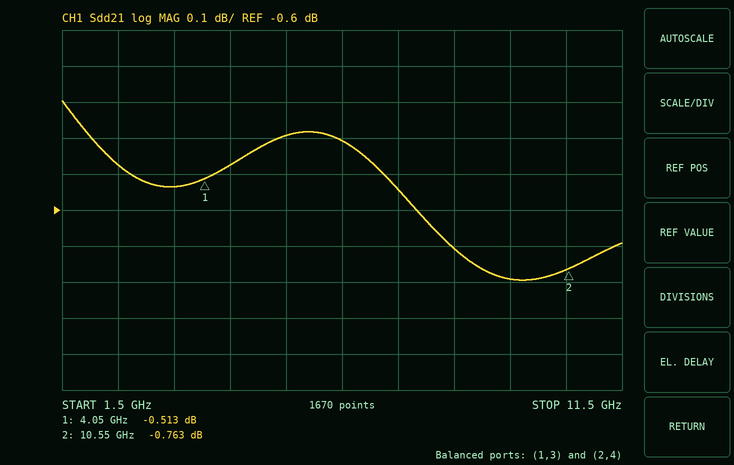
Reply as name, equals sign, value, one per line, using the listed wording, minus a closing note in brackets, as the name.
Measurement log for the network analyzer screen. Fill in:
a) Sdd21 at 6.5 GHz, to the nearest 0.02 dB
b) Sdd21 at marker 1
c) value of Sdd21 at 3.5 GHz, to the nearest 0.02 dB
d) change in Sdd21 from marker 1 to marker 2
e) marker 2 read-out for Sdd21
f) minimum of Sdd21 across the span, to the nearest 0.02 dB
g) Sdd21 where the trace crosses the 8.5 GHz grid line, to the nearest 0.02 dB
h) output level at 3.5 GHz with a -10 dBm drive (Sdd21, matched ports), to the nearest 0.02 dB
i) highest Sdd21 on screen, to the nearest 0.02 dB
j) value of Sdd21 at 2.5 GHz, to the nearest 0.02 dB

Sdd21 at 6.5 GHz, to the nearest 0.02 dB = -0.40 dB
Sdd21 at marker 1 = -0.513 dB
value of Sdd21 at 3.5 GHz, to the nearest 0.02 dB = -0.54 dB
change in Sdd21 from marker 1 to marker 2 = -0.250 dB
marker 2 read-out for Sdd21 = -0.763 dB
minimum of Sdd21 across the span, to the nearest 0.02 dB = -0.80 dB
Sdd21 where the trace crosses the 8.5 GHz grid line, to the nearest 0.02 dB = -0.70 dB
output level at 3.5 GHz with a -10 dBm drive (Sdd21, matched ports), to the nearest 0.02 dB = -10.54 dBm
highest Sdd21 on screen, to the nearest 0.02 dB = -0.30 dB
value of Sdd21 at 2.5 GHz, to the nearest 0.02 dB = -0.48 dB
